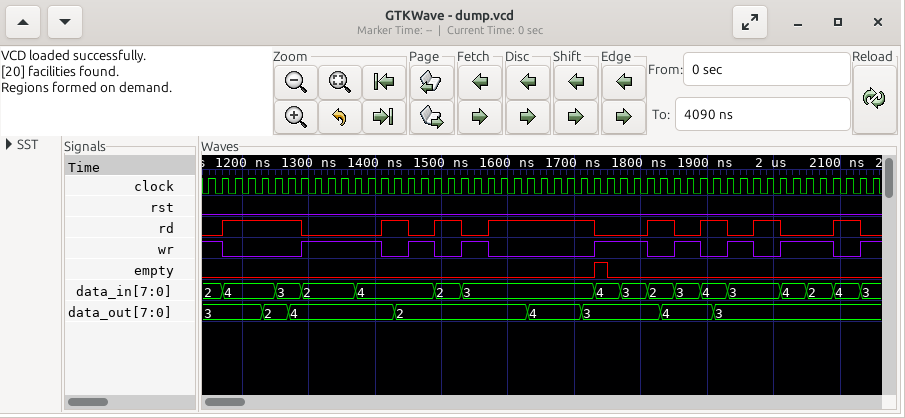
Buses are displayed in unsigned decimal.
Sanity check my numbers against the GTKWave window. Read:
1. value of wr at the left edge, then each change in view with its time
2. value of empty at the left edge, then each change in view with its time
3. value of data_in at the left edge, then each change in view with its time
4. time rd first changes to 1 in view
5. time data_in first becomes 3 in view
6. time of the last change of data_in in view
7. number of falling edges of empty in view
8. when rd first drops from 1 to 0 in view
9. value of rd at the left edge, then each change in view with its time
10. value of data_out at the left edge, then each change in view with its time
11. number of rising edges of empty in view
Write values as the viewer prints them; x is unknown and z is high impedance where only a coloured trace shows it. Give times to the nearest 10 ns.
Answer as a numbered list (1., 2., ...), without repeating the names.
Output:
1. 1, 0 at 1170 ns, 1 at 1290 ns, 0 at 1410 ns, 1 at 1450 ns, 0 at 1490 ns, 1 at 1530 ns, 0 at 1570 ns, 1 at 1730 ns, 0 at 1810 ns, 1 at 1850 ns, 0 at 1890 ns, 1 at 1930 ns, 0 at 1970 ns, 1 at 2010 ns, 0 at 2090 ns, 1 at 2130 ns
2. 0, 1 at 1730 ns, 0 at 1750 ns
3. 2, 4 at 1170 ns, 3 at 1250 ns, 2 at 1290 ns, 4 at 1370 ns, 2 at 1490 ns, 3 at 1530 ns, 4 at 1730 ns, 3 at 1770 ns, 2 at 1810 ns, 3 at 1850 ns, 4 at 1890 ns, 3 at 1930 ns, 4 at 2010 ns, 2 at 2050 ns, 4 at 2090 ns, 3 at 2130 ns
4. 1170 ns
5. 1250 ns
6. 2130 ns
7. 1
8. 1290 ns
9. 0, 1 at 1170 ns, 0 at 1290 ns, 1 at 1410 ns, 0 at 1450 ns, 1 at 1490 ns, 0 at 1530 ns, 1 at 1570 ns, 0 at 1730 ns, 1 at 1810 ns, 0 at 1850 ns, 1 at 1890 ns, 0 at 1930 ns, 1 at 1970 ns, 0 at 2010 ns, 1 at 2090 ns, 0 at 2130 ns
10. 3, 2 at 1230 ns, 4 at 1270 ns, 2 at 1430 ns, 4 at 1630 ns, 3 at 1710 ns, 4 at 1830 ns, 3 at 1910 ns
11. 1
